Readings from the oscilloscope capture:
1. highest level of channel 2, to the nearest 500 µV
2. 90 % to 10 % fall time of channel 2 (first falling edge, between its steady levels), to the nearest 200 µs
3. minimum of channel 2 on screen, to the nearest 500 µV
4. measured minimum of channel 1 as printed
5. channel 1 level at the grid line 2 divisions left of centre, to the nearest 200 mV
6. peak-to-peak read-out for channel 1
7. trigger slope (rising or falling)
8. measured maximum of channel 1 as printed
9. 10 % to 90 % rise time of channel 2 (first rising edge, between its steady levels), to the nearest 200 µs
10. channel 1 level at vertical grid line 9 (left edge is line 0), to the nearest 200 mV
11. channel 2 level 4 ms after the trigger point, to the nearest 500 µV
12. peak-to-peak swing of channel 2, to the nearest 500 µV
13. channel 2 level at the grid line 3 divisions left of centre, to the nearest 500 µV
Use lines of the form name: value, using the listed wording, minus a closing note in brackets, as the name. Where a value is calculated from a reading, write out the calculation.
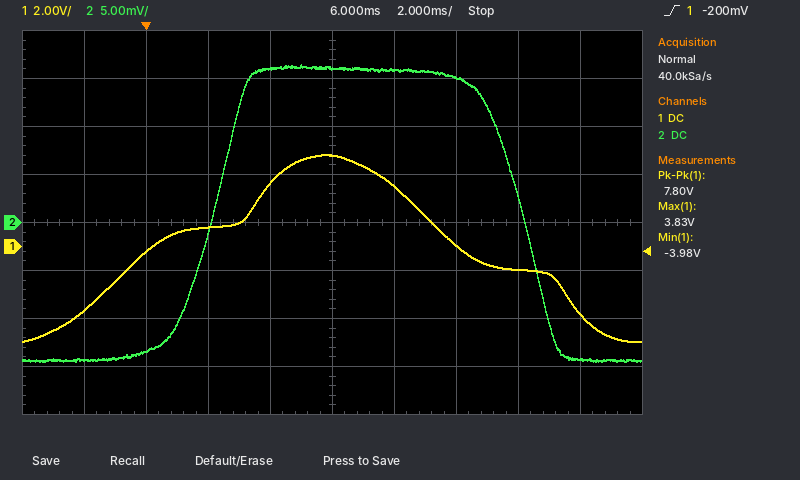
highest level of channel 2, to the nearest 500 µV: 16.5 mV
90 % to 10 % fall time of channel 2 (first falling edge, between its steady levels), to the nearest 200 µs: 2.2 ms
minimum of channel 2 on screen, to the nearest 500 µV: -14.5 mV
measured minimum of channel 1 as printed: -3.98 V
channel 1 level at the grid line 2 divisions left of centre, to the nearest 200 mV: 800 mV
peak-to-peak read-out for channel 1: 7.80 V
trigger slope: rising
measured maximum of channel 1 as printed: 3.83 V
10 % to 90 % rise time of channel 2 (first rising edge, between its steady levels), to the nearest 200 µs: 2.2 ms
channel 1 level at vertical grid line 9 (left edge is line 0), to the nearest 200 mV: -2.8 V
channel 2 level 4 ms after the trigger point, to the nearest 500 µV: 16.0 mV
peak-to-peak swing of channel 2, to the nearest 500 µV: 16.5 mV − (-14.5 mV) = 31.0 mV
channel 2 level at the grid line 3 divisions left of centre, to the nearest 500 µV: -13.5 mV
